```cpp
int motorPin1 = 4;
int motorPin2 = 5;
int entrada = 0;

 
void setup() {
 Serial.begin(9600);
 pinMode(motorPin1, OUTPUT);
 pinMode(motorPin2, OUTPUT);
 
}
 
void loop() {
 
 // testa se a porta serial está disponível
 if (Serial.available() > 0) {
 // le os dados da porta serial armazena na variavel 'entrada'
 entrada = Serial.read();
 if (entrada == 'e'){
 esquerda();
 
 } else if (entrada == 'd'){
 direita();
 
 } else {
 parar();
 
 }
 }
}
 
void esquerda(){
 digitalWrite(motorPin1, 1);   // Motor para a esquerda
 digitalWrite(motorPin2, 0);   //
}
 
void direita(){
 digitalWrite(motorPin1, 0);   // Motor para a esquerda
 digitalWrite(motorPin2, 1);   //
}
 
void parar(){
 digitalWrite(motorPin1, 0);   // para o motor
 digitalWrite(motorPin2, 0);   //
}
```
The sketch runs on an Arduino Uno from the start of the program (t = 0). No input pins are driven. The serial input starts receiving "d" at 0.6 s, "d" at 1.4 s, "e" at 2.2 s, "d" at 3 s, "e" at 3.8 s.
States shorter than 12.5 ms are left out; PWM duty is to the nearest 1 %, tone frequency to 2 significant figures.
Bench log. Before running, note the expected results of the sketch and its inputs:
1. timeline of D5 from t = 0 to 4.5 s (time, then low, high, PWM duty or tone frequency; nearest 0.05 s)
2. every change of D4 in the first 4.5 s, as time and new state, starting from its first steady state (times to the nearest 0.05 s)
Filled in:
0 s low; 0.6 s high; 2.2 s low; 3 s high; 3.8 s low
0 s low; 2.2 s high; 3 s low; 3.8 s high
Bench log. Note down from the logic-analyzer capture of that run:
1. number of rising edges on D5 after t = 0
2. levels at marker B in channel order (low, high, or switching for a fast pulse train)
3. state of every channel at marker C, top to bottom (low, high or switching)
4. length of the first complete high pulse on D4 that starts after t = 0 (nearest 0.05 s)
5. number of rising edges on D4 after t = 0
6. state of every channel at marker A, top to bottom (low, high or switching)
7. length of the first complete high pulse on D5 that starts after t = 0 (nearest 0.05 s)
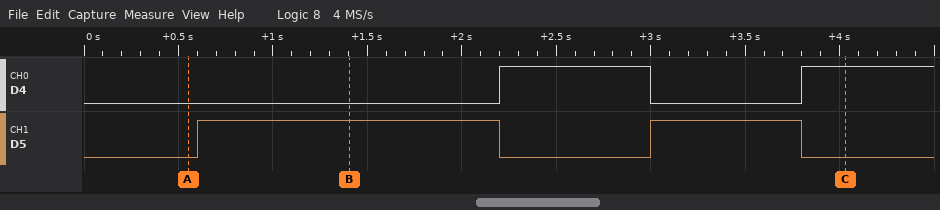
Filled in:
2
D4 low, D5 high
D4 high, D5 low
0.80 s
2
D4 low, D5 low
1.60 s
